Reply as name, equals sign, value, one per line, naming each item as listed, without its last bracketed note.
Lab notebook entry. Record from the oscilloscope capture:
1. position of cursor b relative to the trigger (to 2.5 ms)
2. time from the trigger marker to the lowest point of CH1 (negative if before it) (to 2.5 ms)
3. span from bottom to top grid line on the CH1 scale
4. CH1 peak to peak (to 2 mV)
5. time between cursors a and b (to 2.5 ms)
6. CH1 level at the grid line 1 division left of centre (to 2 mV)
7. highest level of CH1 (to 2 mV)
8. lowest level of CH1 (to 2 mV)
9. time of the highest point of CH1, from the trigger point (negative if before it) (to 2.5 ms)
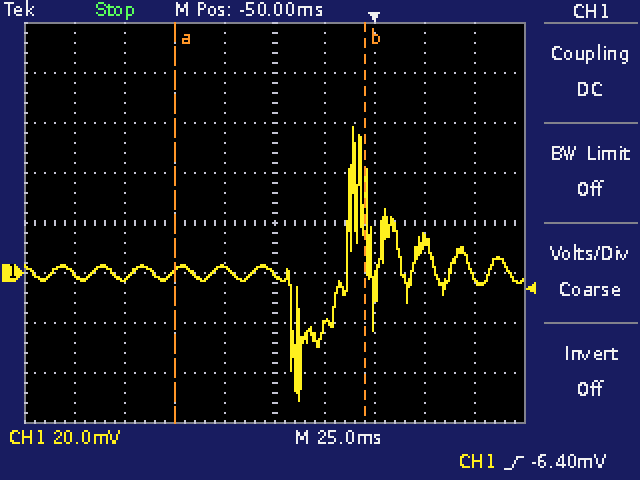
position of cursor b relative to the trigger = -5.0 ms
time from the trigger marker to the lowest point of CH1 (negative if before it) = -37.5 ms
span from bottom to top grid line on the CH1 scale = 160 mV
CH1 peak to peak = 110 mV
time between cursors a and b = 95.0 ms
CH1 level at the grid line 1 division left of centre = 2 mV
highest level of CH1 = 58 mV
lowest level of CH1 = -52 mV
time of the highest point of CH1, from the trigger point (negative if before it) = -10.0 ms
